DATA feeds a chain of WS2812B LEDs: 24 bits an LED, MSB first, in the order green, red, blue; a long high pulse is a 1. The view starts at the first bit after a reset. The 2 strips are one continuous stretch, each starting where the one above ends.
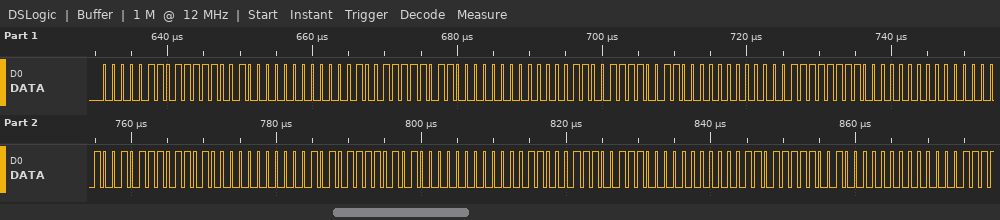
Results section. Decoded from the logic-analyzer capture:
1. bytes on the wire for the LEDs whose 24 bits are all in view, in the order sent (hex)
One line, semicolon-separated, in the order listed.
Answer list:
06 F9 00 09 F6 00 0C F3 00 0F F0 00 12 ED 00 15 EA 00 18 E7 00 1B E4 00
